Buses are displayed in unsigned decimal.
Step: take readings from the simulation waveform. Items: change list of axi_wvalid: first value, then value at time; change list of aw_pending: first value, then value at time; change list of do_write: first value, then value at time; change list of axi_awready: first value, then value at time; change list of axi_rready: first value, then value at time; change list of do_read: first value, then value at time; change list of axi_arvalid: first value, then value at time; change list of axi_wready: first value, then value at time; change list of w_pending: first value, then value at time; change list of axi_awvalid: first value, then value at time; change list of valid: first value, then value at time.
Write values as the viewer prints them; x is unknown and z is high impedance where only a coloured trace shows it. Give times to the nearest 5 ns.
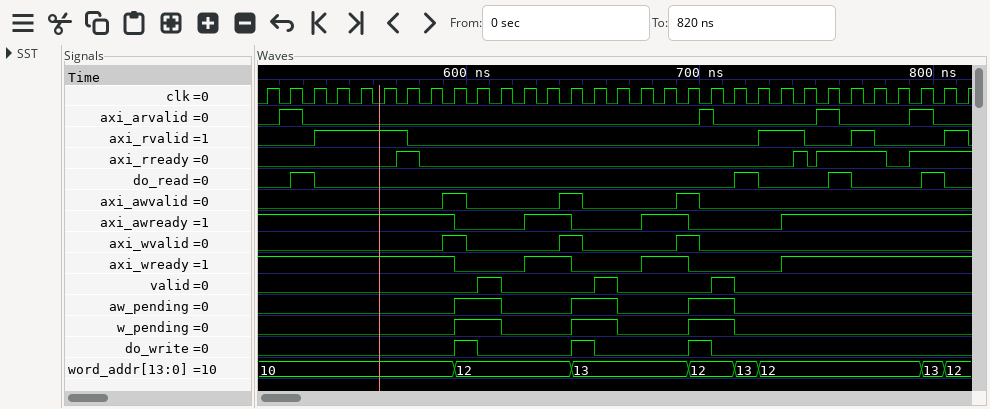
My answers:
0, 1 at 590 ns, 0 at 600 ns, 1 at 640 ns, 0 at 650 ns, 1 at 690 ns, 0 at 700 ns
0, 1 at 595 ns, 0 at 615 ns, 1 at 645 ns, 0 at 665 ns, 1 at 695 ns, 0 at 715 ns
0, 1 at 595 ns, 0 at 605 ns, 1 at 645 ns, 0 at 655 ns, 1 at 695 ns, 0 at 705 ns
1, 0 at 595 ns, 1 at 625 ns, 0 at 645 ns, 1 at 675 ns, 0 at 695 ns, 1 at 735 ns
0, 1 at 570 ns, 0 at 580 ns, 1 at 740 ns, 0 at 745 ns, 1 at 750 ns, 0 at 780 ns, 1 at 790 ns
0, 1 at 525 ns, 0 at 535 ns, 1 at 715 ns, 0 at 725 ns, 1 at 755 ns, 0 at 765 ns, 1 at 795 ns, 0 at 805 ns
0, 1 at 520 ns, 0 at 530 ns, 1 at 700 ns, 0 at 705 ns, 1 at 750 ns, 0 at 760 ns, 1 at 790 ns, 0 at 800 ns
1, 0 at 595 ns, 1 at 625 ns, 0 at 645 ns, 1 at 675 ns, 0 at 695 ns, 1 at 735 ns
0, 1 at 595 ns, 0 at 615 ns, 1 at 645 ns, 0 at 665 ns, 1 at 695 ns, 0 at 715 ns
0, 1 at 590 ns, 0 at 600 ns, 1 at 640 ns, 0 at 650 ns, 1 at 690 ns, 0 at 700 ns
0, 1 at 605 ns, 0 at 615 ns, 1 at 655 ns, 0 at 665 ns, 1 at 705 ns, 0 at 715 ns
